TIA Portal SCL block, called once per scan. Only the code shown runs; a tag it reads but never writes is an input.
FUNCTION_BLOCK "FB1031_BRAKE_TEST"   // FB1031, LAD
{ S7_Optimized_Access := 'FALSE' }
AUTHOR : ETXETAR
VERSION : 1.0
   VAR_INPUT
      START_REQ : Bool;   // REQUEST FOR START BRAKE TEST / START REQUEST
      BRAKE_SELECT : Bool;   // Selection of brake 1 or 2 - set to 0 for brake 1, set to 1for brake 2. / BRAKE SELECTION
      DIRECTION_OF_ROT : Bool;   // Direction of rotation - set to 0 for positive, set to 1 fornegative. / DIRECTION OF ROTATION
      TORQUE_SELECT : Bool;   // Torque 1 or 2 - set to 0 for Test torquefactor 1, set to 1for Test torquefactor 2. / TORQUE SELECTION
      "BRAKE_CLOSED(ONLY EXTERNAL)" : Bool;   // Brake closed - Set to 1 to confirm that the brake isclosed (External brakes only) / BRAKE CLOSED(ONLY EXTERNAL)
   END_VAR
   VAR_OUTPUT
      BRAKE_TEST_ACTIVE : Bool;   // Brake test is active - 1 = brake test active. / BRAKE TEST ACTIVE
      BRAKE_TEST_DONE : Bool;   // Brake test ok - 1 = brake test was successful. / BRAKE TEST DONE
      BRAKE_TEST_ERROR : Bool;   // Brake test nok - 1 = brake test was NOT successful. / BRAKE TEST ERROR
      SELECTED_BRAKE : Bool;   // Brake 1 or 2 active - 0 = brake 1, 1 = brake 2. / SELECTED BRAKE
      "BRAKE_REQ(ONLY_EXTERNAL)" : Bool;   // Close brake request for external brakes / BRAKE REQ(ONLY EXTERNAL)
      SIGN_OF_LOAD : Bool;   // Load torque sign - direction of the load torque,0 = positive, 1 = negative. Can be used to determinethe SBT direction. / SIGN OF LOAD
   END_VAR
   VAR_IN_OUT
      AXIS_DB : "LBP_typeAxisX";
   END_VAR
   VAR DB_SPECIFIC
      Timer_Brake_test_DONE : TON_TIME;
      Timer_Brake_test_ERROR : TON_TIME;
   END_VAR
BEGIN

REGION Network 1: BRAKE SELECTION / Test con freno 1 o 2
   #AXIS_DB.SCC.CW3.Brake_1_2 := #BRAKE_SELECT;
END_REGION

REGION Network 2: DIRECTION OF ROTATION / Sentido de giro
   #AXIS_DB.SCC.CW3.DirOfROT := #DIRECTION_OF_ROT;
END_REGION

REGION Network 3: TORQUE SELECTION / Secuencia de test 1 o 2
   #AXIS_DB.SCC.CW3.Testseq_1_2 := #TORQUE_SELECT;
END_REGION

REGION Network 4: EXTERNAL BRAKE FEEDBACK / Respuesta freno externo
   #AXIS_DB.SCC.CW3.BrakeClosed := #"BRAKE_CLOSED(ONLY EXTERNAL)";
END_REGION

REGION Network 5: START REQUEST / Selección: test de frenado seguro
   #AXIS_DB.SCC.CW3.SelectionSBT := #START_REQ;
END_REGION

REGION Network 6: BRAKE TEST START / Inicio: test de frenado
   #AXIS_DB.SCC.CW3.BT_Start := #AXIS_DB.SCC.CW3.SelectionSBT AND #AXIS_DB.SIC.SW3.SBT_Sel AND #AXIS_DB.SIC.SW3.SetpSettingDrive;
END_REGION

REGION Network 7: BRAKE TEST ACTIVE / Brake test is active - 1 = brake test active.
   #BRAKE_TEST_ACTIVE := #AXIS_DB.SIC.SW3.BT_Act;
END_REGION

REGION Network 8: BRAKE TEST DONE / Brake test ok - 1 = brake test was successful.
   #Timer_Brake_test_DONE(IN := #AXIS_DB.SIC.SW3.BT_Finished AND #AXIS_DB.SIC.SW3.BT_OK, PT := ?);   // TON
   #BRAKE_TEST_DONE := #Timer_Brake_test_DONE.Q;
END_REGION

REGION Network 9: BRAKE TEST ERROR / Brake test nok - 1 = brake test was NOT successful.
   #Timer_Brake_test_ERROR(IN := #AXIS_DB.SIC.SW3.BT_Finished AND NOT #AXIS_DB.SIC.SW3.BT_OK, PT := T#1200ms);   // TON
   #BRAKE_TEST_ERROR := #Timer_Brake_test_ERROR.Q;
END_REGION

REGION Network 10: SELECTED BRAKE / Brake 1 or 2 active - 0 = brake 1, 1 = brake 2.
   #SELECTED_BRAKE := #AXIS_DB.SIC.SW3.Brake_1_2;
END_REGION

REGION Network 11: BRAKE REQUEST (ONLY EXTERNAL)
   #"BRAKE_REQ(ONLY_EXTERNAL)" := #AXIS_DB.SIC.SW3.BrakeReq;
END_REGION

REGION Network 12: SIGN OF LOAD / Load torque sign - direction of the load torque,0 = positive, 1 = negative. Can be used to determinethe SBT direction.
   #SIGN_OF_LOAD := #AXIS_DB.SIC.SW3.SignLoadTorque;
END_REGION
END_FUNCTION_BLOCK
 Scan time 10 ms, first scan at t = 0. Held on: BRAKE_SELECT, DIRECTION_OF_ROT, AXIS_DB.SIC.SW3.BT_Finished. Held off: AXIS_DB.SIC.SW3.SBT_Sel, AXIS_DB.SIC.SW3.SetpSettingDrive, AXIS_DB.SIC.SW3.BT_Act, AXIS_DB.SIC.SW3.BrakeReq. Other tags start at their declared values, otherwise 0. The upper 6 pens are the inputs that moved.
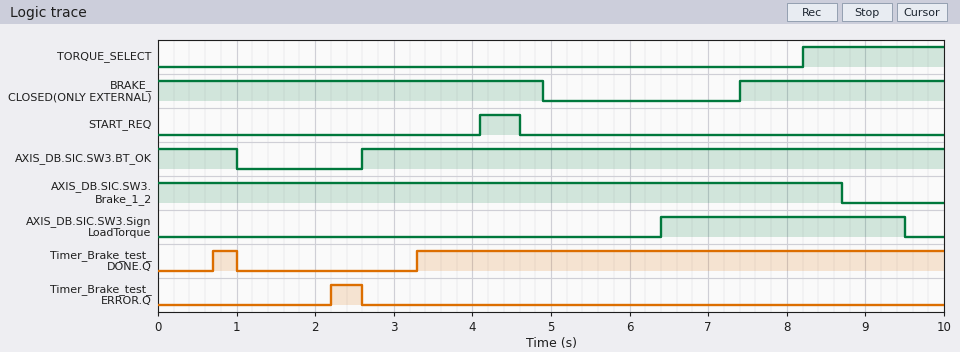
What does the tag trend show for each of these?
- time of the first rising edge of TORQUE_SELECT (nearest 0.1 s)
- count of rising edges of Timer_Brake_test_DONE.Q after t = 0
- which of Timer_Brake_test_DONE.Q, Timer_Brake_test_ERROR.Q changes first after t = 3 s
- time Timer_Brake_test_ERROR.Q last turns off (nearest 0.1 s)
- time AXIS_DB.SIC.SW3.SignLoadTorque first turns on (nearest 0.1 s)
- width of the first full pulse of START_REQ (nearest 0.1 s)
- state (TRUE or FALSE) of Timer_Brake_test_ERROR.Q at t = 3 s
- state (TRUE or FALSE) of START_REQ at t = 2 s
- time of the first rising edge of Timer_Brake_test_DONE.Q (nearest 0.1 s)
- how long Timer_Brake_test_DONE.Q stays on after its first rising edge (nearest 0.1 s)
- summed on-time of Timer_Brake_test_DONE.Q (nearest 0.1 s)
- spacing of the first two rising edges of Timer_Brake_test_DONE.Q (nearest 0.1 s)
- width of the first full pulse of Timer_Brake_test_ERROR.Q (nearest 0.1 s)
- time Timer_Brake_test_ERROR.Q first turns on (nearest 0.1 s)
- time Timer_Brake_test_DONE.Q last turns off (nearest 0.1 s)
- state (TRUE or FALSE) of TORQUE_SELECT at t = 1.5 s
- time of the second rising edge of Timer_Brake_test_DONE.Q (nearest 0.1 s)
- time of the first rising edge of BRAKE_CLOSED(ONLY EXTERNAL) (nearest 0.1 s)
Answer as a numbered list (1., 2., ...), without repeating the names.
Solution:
1. 8.2 s
2. 2
3. Timer_Brake_test_DONE.Q
4. 2.6 s
5. 6.4 s
6. 0.5 s
7. FALSE
8. FALSE
9. 0.7 s
10. 0.3 s
11. 7.0 s
12. 2.6 s
13. 0.4 s
14. 2.2 s
15. 1.0 s
16. FALSE
17. 3.3 s
18. 7.4 s
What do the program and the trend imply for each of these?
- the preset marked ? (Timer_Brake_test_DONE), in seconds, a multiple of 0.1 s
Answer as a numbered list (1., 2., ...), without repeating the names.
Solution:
1. 0.7 s
